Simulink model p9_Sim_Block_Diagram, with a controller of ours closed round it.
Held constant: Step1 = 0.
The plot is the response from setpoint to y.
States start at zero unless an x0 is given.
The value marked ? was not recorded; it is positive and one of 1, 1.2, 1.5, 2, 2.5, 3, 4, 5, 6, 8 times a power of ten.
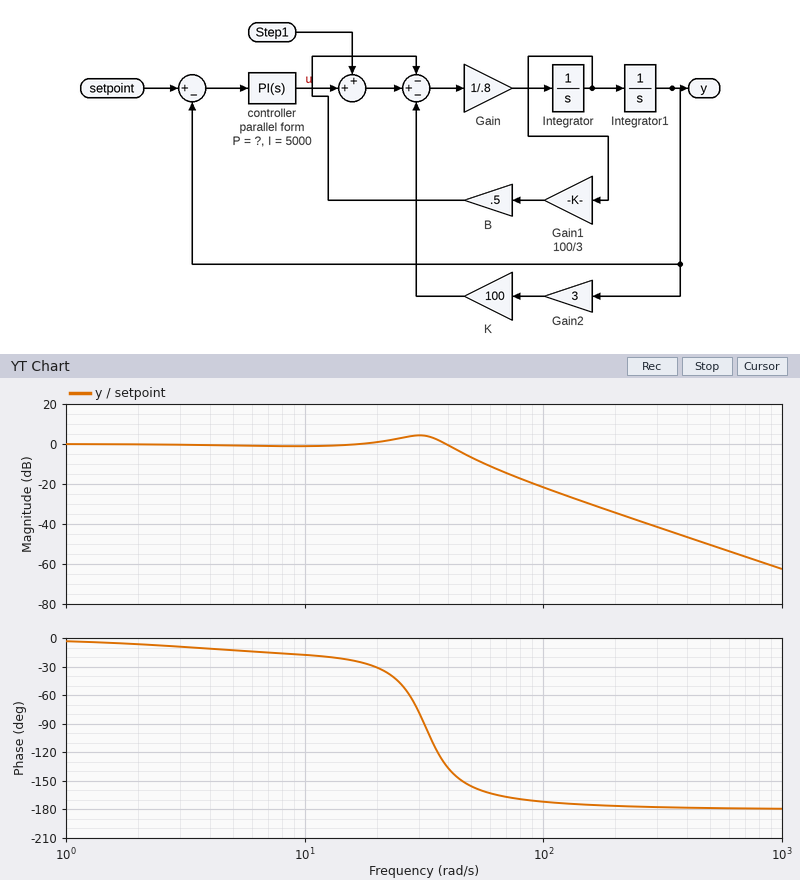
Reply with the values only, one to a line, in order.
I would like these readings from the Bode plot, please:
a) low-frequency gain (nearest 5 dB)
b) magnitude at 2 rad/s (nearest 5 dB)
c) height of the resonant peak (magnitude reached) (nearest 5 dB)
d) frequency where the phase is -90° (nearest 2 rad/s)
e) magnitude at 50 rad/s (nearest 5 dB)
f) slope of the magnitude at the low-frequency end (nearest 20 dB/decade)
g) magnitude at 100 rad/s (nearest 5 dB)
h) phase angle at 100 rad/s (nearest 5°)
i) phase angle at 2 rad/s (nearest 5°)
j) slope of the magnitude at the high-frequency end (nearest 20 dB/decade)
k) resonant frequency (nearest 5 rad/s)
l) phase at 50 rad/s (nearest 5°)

0 dB
0 dB
5 dB
32 rad/s
-5 dB
0 dB/decade
-20 dB
-170°
-5°
-40 dB/decade
30 rad/s
-155°
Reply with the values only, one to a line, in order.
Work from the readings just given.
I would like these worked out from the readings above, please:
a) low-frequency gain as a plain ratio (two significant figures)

1.0
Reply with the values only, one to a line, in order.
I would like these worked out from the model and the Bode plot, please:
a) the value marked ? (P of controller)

600
